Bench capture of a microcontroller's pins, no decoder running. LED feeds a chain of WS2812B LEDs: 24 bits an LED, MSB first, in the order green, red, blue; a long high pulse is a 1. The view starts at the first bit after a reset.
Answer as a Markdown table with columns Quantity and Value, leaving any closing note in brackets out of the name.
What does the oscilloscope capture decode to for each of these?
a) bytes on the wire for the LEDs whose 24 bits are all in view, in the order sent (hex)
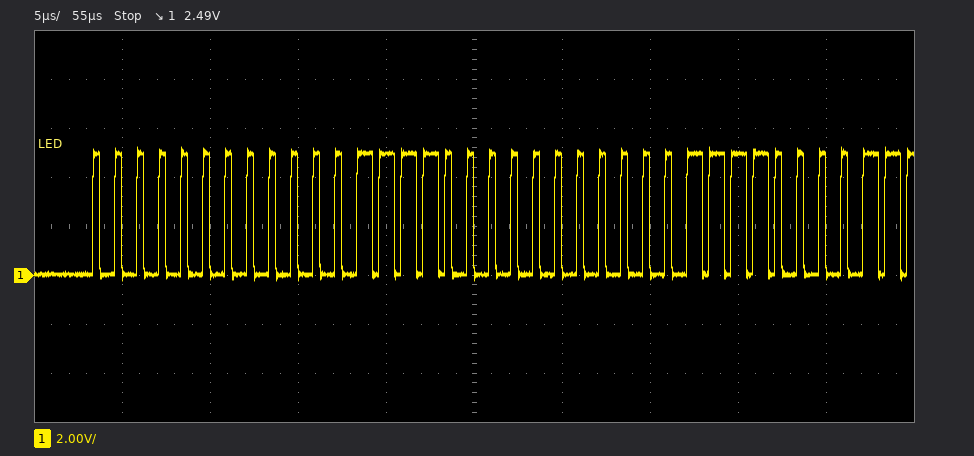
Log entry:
| Quantity | Value |
|---|---|
| bytes on the wire for the LEDs whose 24 bits are all in view, in the order sent | 00 0F 00 |
